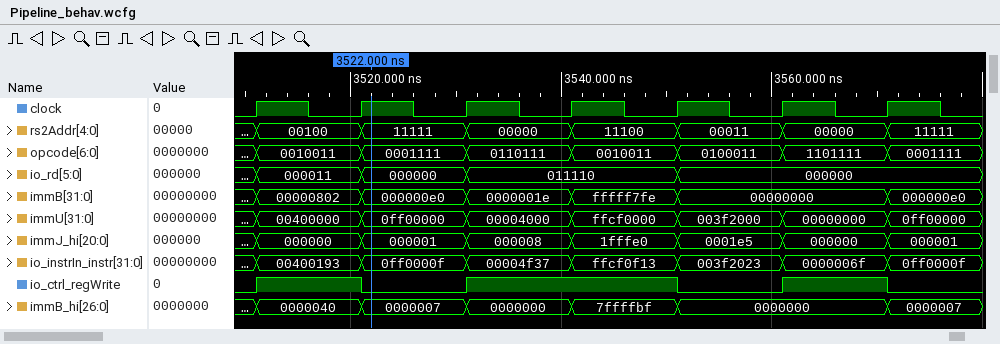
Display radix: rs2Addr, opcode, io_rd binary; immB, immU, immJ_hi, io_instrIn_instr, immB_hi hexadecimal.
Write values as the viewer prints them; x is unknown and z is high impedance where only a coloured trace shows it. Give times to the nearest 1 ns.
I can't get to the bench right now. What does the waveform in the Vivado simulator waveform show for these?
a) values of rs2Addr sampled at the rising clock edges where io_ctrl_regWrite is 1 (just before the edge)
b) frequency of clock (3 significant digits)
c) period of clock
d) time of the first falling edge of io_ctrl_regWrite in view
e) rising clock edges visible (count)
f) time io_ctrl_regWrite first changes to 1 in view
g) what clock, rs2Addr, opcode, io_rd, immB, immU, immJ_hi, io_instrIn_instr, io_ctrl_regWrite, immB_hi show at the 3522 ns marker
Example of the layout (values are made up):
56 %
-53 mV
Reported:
00100, 00000, 11100, 00000
100 MHz
10 ns
3521 ns
7
3511 ns
clock=1, rs2Addr=11111, opcode=0001111, io_rd=000000, immB=000000e0, immU=0ff00000, immJ_hi=000001, io_instrIn_instr=0ff0000f, io_ctrl_regWrite=0, immB_hi=0000007
